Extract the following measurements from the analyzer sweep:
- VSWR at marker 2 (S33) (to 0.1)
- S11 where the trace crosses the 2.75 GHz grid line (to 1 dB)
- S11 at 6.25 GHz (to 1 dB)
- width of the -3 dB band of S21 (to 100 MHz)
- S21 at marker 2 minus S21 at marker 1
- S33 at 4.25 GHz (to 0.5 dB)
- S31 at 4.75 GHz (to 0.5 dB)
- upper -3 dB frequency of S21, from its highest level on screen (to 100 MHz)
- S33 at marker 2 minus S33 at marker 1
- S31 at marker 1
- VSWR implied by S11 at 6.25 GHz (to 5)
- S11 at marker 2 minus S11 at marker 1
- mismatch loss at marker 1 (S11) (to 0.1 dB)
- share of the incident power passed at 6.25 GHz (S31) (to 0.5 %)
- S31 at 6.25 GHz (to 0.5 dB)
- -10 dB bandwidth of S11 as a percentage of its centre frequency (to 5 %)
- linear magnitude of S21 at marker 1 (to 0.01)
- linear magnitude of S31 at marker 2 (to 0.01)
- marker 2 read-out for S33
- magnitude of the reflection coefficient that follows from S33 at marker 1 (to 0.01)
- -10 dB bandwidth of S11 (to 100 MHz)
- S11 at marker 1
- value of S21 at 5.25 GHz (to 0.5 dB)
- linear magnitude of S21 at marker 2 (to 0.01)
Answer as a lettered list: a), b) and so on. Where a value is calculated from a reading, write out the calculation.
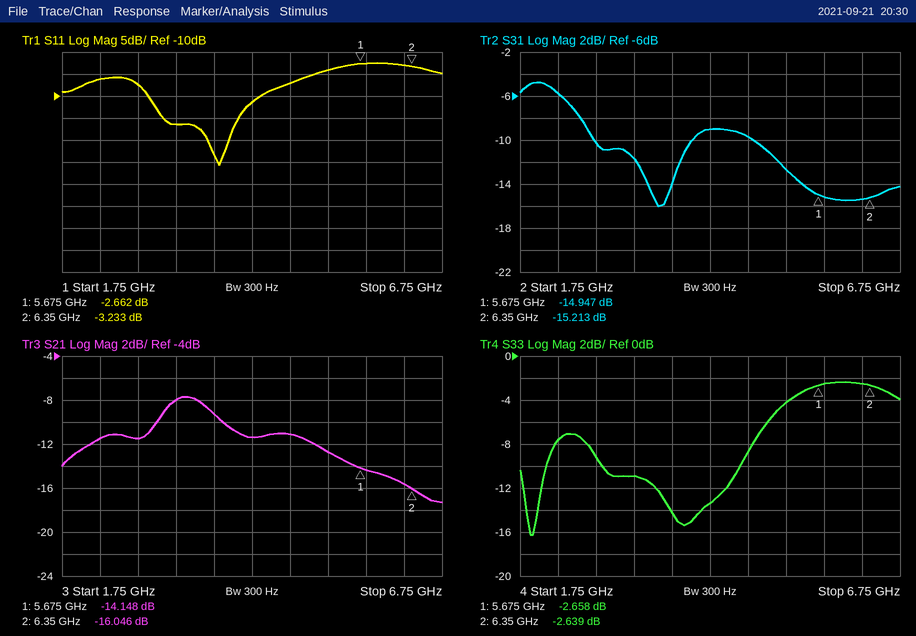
a) (1 + 0.7380)/(1 − 0.7380) ≈ 6.6
b) -7 dB
c) -3 dB
d) 4.0 GHz − 2.9 GHz = 1.1 GHz
e) -16.046 − (-14.148) = -1.898 dB
f) -13.5 dB
g) -9.5 dB
h) 4.0 GHz
i) -2.639 − (-2.658) = 0.019 dB
j) -14.947 dB
k) |Γ| = 10^(-3/20) = 0.7079; VSWR = (1 + 0.7079)/(1 − 0.7079) ≈ 5.85, so 5 to the nearest 5
l) -3.233 − (-2.662) = -0.571 dB
m) −10 log10(1 − 10^(-2.662/10)) ≈ 3.4 dB
n) 10^(-15.5/10) ≈ 2.82 %, so 3.0 % to the nearest 0.5 %
o) -15.5 dB
p) 1.5 GHz / 3.65 GHz ≈ 41.1 %, so 40 % to the nearest 5 %
q) 10^(-14.148/20) ≈ 0.20
r) 10^(-15.213/20) ≈ 0.17
s) -2.639 dB
t) 10^(-2.658/20) ≈ 0.74
u) 4.4 GHz − 2.9 GHz = 1.5 GHz
v) -2.662 dB
w) -12.5 dB
x) 10^(-16.046/20) ≈ 0.16
